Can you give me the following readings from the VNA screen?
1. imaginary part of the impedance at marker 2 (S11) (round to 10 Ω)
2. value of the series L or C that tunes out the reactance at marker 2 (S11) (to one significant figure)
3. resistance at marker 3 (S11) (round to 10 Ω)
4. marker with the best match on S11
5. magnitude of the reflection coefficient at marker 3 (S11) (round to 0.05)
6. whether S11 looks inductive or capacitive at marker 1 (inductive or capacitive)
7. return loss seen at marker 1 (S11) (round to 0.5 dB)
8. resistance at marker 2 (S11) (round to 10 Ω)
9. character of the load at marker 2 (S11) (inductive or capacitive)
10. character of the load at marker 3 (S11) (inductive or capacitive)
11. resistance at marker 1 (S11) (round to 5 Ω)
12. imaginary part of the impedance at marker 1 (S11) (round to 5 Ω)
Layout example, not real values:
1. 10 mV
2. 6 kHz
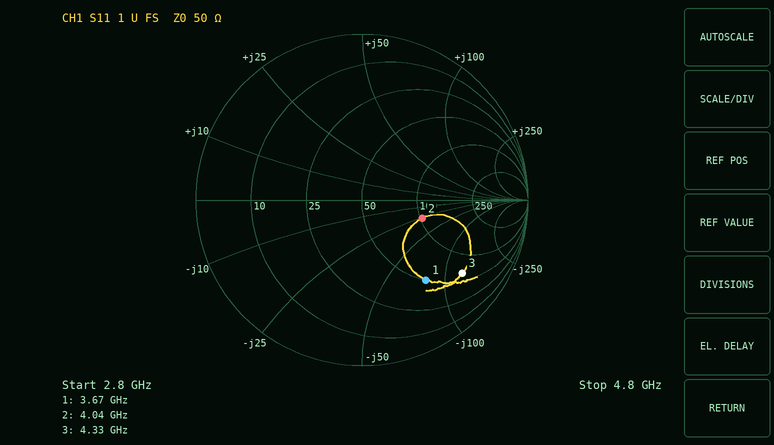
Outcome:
1. -30 Ω
2. 1 nH
3. 60 Ω
4. marker 2
5. 0.75
6. capacitive
7. 4.0 dB
8. 100 Ω
9. capacitive
10. capacitive
11. 50 Ω
12. -80 Ω
